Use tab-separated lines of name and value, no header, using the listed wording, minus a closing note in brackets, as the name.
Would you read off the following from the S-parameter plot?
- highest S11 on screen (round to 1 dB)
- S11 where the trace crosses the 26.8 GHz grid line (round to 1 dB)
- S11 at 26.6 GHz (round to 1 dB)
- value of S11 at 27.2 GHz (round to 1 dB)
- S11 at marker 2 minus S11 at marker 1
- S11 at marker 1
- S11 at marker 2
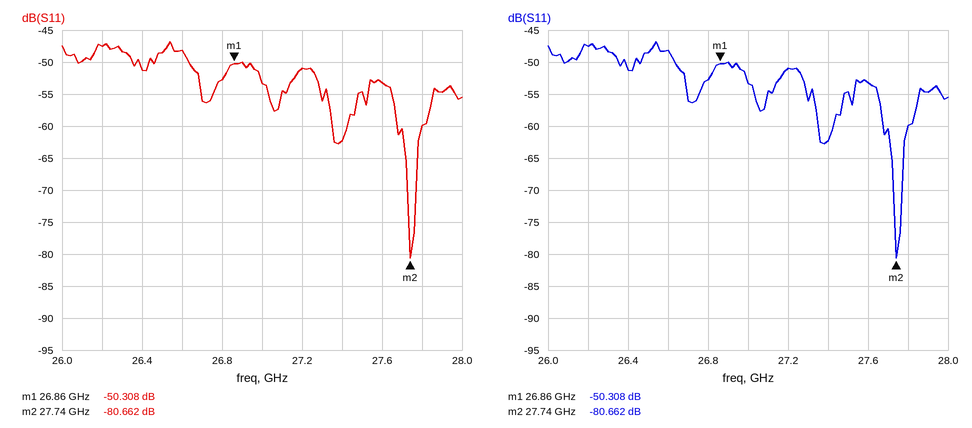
highest S11 on screen	-47 dB
S11 where the trace crosses the 26.8 GHz grid line	-53 dB
S11 at 26.6 GHz	-48 dB
value of S11 at 27.2 GHz	-51 dB
S11 at marker 2 minus S11 at marker 1	-30.354 dB
S11 at marker 1	-50.308 dB
S11 at marker 2	-80.662 dB
